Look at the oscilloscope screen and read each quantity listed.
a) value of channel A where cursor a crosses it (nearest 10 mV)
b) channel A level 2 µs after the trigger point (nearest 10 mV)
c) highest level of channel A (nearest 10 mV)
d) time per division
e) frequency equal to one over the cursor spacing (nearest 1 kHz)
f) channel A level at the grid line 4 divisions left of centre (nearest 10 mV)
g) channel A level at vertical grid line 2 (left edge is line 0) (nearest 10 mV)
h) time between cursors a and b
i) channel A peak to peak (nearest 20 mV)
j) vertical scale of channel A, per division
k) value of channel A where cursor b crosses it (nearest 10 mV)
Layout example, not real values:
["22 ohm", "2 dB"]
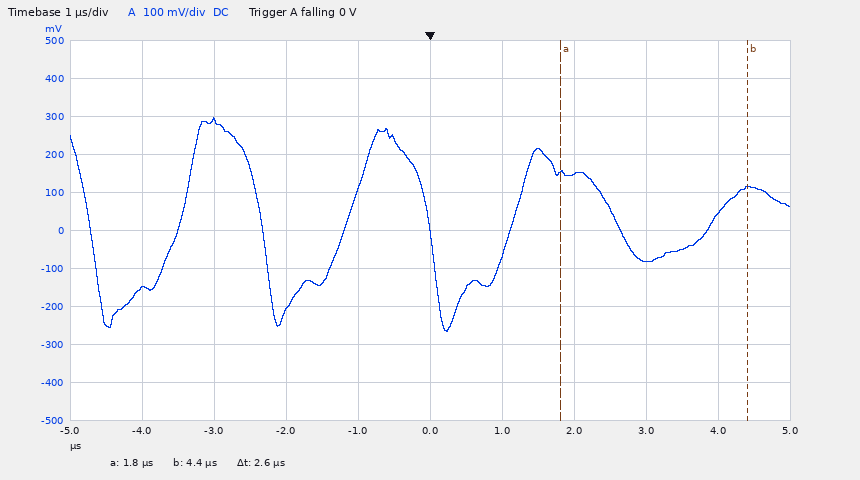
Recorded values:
["150 mV", "150 mV", "300 mV", "1 µs", "385 kHz", "-150 mV", "290 mV", "2.6 µs", "560 mV", "100 mV", "110 mV"]
